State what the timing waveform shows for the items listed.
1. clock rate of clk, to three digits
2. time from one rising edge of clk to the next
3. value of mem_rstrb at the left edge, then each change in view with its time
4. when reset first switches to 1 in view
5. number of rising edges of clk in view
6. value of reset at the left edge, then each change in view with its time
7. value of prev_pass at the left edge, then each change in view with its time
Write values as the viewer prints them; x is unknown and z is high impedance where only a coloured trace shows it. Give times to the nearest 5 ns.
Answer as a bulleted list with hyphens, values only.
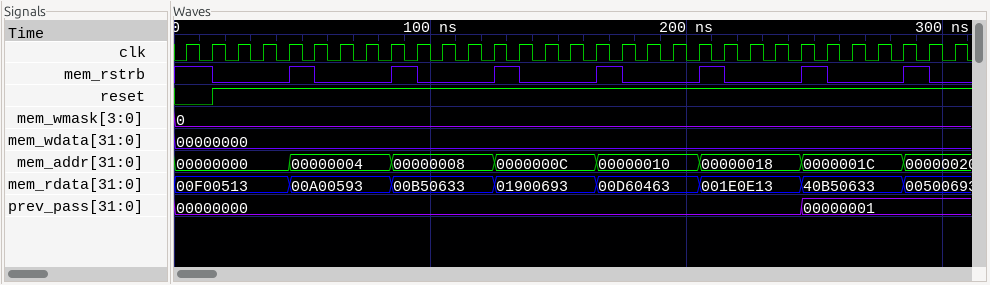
- 100 MHz
- 10 ns
- 1, 0 at 15 ns, 1 at 45 ns, 0 at 55 ns, 1 at 85 ns, 0 at 95 ns, 1 at 125 ns, 0 at 135 ns, 1 at 165 ns, 0 at 175 ns, 1 at 205 ns, 0 at 215 ns, 1 at 245 ns, 0 at 255 ns, 1 at 285 ns, 0 at 295 ns
- 15 ns
- 31
- 0, 1 at 15 ns
- 00000000, 00000001 at 245 ns
